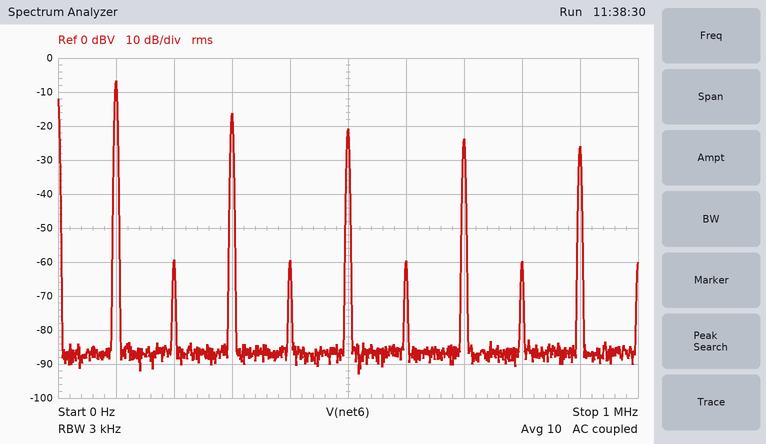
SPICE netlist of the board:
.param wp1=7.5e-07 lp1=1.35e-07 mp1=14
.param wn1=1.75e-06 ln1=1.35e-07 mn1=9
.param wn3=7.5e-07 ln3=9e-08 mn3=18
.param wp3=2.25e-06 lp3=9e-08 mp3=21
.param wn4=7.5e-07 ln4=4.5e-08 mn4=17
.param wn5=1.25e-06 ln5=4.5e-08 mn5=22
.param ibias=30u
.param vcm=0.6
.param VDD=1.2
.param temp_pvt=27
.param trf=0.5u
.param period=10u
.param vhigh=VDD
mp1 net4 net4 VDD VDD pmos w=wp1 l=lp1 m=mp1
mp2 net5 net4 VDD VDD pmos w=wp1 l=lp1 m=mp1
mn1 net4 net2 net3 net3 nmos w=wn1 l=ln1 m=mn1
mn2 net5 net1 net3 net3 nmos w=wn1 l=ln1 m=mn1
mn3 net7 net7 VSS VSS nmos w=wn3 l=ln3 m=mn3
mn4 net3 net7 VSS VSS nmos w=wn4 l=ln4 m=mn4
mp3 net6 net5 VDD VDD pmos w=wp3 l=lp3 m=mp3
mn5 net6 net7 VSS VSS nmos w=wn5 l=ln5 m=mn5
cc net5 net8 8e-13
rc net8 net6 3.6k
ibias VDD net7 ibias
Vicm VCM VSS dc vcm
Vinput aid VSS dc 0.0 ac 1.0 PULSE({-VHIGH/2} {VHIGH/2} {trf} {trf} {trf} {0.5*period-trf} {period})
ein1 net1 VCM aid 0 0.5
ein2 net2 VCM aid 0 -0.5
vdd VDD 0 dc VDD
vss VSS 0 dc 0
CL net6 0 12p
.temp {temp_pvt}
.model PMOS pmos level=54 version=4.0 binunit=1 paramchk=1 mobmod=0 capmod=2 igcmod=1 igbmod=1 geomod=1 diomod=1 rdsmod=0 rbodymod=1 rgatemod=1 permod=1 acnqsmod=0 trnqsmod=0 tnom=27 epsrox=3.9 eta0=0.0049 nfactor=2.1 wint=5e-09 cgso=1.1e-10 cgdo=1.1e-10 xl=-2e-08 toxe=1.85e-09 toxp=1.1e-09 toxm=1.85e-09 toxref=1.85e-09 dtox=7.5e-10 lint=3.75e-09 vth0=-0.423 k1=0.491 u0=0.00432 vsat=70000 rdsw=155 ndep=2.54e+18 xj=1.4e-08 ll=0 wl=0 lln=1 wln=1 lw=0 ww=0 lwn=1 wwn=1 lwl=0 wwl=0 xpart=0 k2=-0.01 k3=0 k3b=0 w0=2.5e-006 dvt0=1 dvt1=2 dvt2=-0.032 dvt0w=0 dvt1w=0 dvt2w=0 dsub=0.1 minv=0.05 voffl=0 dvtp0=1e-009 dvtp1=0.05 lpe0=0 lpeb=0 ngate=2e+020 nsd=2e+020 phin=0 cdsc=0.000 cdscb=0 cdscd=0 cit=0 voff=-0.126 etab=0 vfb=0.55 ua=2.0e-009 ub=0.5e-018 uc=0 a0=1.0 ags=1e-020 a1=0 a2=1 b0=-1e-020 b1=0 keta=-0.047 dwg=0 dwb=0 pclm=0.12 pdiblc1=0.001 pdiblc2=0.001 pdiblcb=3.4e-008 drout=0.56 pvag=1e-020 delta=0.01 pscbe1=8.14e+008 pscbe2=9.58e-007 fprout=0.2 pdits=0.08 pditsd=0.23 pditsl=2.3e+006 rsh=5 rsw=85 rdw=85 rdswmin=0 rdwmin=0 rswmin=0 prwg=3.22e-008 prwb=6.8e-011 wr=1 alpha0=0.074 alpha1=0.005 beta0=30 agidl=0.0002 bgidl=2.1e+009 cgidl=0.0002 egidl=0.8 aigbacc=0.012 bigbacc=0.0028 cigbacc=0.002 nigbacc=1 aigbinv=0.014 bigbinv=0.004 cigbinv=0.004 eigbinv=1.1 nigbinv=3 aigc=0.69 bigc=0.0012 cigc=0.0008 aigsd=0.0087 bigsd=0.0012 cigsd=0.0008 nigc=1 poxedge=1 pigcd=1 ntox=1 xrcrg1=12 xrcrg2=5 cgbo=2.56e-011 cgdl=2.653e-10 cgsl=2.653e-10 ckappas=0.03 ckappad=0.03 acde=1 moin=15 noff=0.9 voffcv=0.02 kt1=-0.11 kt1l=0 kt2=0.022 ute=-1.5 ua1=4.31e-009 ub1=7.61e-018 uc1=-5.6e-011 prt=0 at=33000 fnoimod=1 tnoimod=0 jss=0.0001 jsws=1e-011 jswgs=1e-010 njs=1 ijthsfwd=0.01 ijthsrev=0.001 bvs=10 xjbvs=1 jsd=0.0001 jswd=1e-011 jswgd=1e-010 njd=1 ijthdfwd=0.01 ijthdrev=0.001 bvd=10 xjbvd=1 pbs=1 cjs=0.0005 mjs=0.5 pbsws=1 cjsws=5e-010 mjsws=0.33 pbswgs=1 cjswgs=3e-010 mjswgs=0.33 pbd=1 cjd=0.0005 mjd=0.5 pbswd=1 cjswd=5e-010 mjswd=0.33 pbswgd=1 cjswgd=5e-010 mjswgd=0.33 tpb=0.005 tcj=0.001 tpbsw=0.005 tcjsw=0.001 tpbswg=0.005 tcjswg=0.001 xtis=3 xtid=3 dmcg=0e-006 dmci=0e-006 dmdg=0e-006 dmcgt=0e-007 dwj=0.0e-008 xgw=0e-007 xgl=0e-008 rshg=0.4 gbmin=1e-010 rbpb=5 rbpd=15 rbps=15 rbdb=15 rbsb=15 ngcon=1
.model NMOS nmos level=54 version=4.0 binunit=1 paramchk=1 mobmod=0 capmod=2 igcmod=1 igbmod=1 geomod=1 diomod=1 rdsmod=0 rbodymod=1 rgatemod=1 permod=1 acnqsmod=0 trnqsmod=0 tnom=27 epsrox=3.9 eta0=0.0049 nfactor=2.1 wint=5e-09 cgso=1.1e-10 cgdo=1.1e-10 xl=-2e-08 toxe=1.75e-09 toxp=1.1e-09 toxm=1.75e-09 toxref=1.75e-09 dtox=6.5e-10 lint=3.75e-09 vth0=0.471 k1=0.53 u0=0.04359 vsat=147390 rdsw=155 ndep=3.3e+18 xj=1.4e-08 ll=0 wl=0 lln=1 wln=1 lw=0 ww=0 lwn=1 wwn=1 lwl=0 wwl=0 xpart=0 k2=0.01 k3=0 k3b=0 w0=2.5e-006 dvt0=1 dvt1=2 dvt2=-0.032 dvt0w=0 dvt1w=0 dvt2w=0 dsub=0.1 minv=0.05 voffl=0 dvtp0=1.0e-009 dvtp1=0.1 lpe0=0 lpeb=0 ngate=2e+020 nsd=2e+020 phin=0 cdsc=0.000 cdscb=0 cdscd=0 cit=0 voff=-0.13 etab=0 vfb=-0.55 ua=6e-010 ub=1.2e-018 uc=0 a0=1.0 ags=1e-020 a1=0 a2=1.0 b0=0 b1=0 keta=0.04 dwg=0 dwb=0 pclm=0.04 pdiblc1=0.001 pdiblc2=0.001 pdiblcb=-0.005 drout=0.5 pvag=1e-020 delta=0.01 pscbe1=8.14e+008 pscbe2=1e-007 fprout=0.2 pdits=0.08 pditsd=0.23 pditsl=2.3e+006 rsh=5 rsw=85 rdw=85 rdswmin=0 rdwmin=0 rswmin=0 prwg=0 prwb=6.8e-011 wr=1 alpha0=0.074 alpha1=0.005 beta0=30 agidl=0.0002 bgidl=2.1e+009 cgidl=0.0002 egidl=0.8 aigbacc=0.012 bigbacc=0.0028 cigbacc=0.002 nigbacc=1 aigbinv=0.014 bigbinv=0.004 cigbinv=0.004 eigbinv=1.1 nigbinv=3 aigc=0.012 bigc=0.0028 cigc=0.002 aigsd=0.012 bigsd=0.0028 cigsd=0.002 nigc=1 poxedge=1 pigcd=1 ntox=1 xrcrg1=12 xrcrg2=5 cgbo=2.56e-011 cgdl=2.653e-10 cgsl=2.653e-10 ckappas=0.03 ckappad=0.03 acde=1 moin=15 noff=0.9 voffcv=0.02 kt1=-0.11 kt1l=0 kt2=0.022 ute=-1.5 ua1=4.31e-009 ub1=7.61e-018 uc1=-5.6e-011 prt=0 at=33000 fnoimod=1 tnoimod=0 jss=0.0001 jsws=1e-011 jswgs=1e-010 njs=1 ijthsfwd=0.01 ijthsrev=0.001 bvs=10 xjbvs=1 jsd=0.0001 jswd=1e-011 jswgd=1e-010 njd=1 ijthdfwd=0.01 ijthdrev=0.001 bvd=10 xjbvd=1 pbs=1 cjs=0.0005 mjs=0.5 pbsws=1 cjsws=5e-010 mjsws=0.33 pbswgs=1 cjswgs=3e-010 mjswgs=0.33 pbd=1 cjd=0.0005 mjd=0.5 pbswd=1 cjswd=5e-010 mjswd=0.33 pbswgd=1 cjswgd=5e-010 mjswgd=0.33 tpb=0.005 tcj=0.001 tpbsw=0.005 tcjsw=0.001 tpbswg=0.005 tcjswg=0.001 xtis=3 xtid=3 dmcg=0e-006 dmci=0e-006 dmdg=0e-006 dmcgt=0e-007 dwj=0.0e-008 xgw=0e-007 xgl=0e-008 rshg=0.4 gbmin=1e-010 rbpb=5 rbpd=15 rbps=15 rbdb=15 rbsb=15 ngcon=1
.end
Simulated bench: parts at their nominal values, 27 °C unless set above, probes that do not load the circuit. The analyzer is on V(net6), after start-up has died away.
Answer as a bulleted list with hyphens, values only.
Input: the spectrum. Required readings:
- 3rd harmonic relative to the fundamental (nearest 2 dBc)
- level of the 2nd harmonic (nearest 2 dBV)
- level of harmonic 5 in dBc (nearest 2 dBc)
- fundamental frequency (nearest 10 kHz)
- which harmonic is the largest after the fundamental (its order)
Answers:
- -10 dBc
- -60 dBV
- -14 dBc
- 100 kHz
- 3
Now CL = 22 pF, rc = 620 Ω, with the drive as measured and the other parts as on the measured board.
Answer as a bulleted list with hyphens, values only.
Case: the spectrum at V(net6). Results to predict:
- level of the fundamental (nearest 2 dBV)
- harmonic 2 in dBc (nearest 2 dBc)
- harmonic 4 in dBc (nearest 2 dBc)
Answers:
- -6 dBV
- -56 dBc
- -56 dBc
